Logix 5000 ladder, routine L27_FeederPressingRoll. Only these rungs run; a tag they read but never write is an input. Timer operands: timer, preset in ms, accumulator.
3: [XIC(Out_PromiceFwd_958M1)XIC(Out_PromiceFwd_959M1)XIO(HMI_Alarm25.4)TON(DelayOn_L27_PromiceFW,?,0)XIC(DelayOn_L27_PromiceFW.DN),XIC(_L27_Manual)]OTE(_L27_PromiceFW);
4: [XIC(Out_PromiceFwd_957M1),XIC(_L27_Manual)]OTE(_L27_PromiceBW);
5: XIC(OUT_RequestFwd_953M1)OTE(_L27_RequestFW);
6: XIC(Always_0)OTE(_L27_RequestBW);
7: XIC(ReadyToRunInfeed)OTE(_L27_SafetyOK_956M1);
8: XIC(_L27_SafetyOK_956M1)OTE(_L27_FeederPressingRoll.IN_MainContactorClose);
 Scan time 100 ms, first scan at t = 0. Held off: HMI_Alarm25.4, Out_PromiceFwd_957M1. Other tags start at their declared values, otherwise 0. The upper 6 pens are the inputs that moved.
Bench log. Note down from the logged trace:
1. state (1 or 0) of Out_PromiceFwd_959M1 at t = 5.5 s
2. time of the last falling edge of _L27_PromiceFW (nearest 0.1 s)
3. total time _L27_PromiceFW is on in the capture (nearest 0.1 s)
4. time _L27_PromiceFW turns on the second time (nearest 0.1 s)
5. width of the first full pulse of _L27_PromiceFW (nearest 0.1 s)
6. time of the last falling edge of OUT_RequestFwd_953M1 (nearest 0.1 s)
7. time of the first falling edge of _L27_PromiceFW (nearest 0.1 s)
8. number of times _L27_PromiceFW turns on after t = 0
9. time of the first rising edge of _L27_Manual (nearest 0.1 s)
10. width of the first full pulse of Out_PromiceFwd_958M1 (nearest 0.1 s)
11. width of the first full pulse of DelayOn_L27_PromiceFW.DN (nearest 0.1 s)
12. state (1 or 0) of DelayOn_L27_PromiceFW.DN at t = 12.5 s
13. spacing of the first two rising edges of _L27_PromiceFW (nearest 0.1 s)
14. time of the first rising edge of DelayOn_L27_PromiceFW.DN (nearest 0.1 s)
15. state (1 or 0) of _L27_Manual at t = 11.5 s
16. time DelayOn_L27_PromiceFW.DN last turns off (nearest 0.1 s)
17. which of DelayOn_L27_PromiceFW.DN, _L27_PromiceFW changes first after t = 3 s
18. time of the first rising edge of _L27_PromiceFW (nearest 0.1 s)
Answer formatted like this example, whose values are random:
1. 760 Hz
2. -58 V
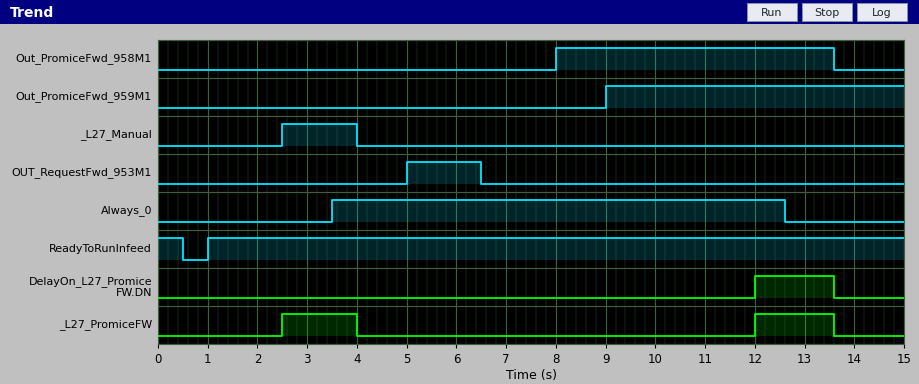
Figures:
1. 0
2. 13.6 s
3. 3.1 s
4. 12.0 s
5. 1.5 s
6. 6.5 s
7. 4.0 s
8. 2
9. 2.5 s
10. 5.6 s
11. 1.6 s
12. 1
13. 9.5 s
14. 12.0 s
15. 0
16. 13.6 s
17. _L27_PromiceFW
18. 2.5 s
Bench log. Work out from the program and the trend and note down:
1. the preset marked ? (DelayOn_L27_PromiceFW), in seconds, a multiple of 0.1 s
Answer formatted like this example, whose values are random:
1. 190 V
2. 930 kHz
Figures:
1. 3.0 s
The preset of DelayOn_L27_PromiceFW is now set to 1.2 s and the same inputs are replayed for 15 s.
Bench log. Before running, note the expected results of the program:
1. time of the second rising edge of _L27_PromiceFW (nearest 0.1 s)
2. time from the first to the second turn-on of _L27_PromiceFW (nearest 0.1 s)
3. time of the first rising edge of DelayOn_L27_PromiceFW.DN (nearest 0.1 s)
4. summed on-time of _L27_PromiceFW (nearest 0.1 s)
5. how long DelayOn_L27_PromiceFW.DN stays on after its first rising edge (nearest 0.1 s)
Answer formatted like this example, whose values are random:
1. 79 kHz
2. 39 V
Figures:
1. 10.2 s
2. 7.7 s
3. 10.2 s
4. 4.9 s
5. 3.4 s
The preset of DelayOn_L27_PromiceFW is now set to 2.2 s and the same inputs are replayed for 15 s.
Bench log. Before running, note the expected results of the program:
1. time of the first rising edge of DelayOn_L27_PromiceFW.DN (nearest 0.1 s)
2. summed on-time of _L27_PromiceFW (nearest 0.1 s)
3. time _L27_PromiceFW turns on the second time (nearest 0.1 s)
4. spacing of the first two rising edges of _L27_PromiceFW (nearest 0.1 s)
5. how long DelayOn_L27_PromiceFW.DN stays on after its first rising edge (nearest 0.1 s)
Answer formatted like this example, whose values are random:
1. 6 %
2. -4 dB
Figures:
1. 11.2 s
2. 3.9 s
3. 11.2 s
4. 8.7 s
5. 2.4 s
